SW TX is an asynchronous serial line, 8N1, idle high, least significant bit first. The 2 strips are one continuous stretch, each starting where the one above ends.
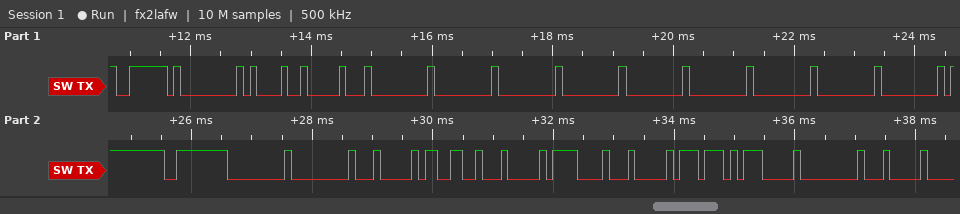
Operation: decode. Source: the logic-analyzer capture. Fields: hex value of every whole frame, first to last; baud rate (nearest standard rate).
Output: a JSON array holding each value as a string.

["0x7E 0x00 0x21 0x10 0x00 0x00 0x00 0x00 0x00 0x00 0x00 0x00 0x00 0xFF 0xFE 0x00 0x00 0x04 0x33 0x04 0x0F 0x04 0x77 0x07 0x00 0x04", "9600 baud"]
